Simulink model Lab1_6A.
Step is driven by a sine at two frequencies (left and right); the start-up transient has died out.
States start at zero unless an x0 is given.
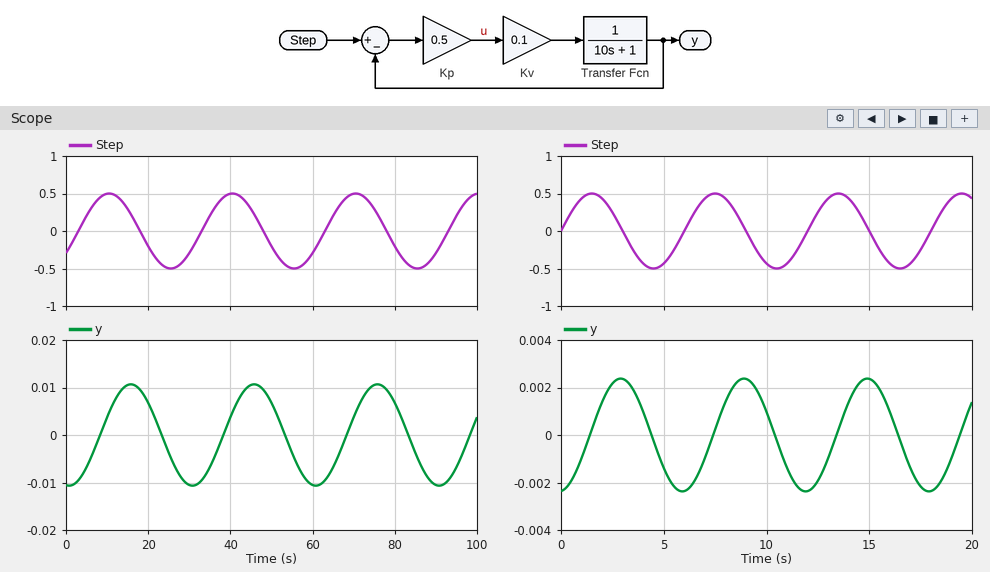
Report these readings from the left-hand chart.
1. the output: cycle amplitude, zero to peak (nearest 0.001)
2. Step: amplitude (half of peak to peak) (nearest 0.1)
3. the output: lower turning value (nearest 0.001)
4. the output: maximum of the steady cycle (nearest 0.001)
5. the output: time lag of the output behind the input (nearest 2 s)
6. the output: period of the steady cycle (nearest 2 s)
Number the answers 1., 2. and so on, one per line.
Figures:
1. 0.011
2. 0.5
3. -0.011
4. 0.011
5. 6 s
6. 30 s
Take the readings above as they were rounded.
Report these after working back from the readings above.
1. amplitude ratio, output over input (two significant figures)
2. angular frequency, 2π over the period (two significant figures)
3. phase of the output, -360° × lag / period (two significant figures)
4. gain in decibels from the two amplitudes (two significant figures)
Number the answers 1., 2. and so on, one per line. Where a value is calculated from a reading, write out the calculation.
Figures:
1. 0.011 / 0.5 = 0.022
2. 2π / 30 = 0.21 rad/s
3. -360 × 6 / 30 = -72°
4. 20 log10(0.011 / 0.5) = -33 dB
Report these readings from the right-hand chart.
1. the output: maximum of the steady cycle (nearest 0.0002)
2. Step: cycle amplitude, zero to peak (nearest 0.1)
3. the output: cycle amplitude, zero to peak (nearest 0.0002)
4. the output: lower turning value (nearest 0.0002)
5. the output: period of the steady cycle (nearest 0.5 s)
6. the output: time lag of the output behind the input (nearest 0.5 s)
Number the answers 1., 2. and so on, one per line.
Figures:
1. 0.0024
2. 0.5
3. 0.0024
4. -0.0024
5. 6.0 s
6. 1.5 s
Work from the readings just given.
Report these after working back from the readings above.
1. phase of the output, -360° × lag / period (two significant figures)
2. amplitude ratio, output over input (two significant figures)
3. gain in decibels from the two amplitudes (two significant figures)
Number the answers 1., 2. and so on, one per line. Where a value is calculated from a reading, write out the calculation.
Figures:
1. -360 × 1.5 / 6 = -90°
2. 0.0024 / 0.5 = 0.0048
3. 20 log10(0.0024 / 0.5) = -46 dB
